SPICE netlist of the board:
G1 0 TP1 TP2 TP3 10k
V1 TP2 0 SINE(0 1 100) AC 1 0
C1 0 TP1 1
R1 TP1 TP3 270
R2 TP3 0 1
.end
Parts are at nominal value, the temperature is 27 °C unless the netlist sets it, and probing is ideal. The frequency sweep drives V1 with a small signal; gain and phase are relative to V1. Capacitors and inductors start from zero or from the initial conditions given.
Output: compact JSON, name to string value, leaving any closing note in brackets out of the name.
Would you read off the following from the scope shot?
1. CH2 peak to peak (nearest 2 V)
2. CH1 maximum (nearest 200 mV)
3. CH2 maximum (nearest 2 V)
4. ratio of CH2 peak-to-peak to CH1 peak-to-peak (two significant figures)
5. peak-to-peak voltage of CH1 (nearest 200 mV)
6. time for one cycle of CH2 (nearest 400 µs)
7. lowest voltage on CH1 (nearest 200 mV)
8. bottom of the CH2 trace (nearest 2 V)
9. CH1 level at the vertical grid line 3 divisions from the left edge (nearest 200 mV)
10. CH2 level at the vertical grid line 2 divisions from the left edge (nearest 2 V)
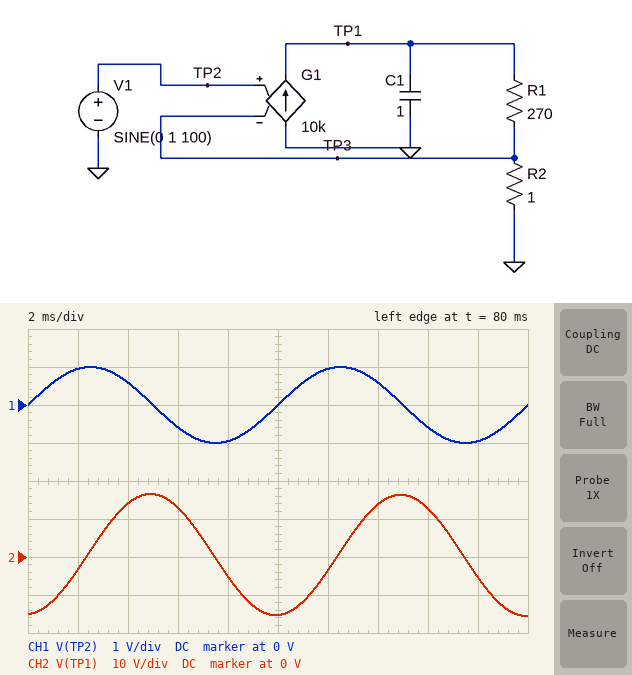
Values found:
{"CH2 peak to peak": "32 V", "CH1 maximum": "1.0 V", "CH2 maximum": "16 V", "ratio of CH2 peak-to-peak to CH1 peak-to-peak": "16", "peak-to-peak voltage of CH1": "2.0 V", "time for one cycle of CH2": "10.0 ms", "lowest voltage on CH1": "-1.0 V", "bottom of the CH2 trace": "-16 V", "CH1 level at the vertical grid line 3 divisions from the left edge": "-600 mV", "CH2 level at the vertical grid line 2 divisions from the left edge": "14 V"}
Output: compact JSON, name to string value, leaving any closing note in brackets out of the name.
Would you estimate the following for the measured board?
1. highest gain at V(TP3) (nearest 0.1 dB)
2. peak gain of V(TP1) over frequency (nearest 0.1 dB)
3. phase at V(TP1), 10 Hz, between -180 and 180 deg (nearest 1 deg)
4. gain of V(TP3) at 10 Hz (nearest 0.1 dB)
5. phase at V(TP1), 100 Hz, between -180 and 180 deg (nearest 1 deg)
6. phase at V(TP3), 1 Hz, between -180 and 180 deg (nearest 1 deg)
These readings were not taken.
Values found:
{"highest gain at V(TP3)": "0 dB", "peak gain of V(TP1) over frequency": "48.7 dB", "phase at V(TP1), 10 Hz, between -180 and 180 deg": "-60 deg", "gain of V(TP3) at 10 Hz": "-5.9 dB", "phase at V(TP1), 100 Hz, between -180 and 180 deg": "-87 deg", "phase at V(TP3), 1 Hz, between -180 and 180 deg": "-10 deg"}
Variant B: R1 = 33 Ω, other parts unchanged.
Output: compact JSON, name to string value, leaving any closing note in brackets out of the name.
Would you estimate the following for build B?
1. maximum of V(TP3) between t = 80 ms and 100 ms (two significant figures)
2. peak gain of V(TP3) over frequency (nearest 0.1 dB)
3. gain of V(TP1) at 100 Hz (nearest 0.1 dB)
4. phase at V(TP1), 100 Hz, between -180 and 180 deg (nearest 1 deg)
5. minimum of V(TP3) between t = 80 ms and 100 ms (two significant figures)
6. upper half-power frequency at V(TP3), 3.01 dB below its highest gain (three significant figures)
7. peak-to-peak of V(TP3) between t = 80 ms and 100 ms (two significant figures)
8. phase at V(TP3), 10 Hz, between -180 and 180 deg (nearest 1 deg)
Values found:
{"maximum of V(TP3) between t = 80 ms and 100 ms": "420 mV", "peak gain of V(TP3) over frequency": "0 dB", "gain of V(TP1) at 100 Hz": "23.2 dB", "phase at V(TP1), 100 Hz, between -180 and 180 deg": "-65 deg", "minimum of V(TP3) between t = 80 ms and 100 ms": "-420 mV", "upper half-power frequency at V(TP3), 3.01 dB below its highest gain": "46.8 Hz", "peak-to-peak of V(TP3) between t = 80 ms and 100 ms": "850 mV", "phase at V(TP3), 10 Hz, between -180 and 180 deg": "-12 deg"}
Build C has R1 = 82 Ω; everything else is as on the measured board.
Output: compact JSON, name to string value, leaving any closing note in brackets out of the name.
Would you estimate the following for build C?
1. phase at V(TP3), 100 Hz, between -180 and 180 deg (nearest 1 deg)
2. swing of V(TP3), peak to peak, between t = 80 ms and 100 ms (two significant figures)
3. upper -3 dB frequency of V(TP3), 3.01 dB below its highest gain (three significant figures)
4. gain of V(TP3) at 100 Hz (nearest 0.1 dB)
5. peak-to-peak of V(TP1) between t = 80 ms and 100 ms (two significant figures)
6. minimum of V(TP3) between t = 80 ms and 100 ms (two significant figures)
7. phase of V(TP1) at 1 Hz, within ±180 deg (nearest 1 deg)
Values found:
{"phase at V(TP3), 100 Hz, between -180 and 180 deg": "-79 deg", "swing of V(TP3), peak to peak, between t = 80 ms and 100 ms": "380 mV", "upper -3 dB frequency of V(TP3), 3.01 dB below its highest gain": "19.2 Hz", "gain of V(TP3) at 100 Hz": "-14.5 dB", "peak-to-peak of V(TP1) between t = 80 ms and 100 ms": "31 V", "minimum of V(TP3) between t = 80 ms and 100 ms": "-190 mV", "phase of V(TP1) at 1 Hz, within ±180 deg": "-3 deg"}
